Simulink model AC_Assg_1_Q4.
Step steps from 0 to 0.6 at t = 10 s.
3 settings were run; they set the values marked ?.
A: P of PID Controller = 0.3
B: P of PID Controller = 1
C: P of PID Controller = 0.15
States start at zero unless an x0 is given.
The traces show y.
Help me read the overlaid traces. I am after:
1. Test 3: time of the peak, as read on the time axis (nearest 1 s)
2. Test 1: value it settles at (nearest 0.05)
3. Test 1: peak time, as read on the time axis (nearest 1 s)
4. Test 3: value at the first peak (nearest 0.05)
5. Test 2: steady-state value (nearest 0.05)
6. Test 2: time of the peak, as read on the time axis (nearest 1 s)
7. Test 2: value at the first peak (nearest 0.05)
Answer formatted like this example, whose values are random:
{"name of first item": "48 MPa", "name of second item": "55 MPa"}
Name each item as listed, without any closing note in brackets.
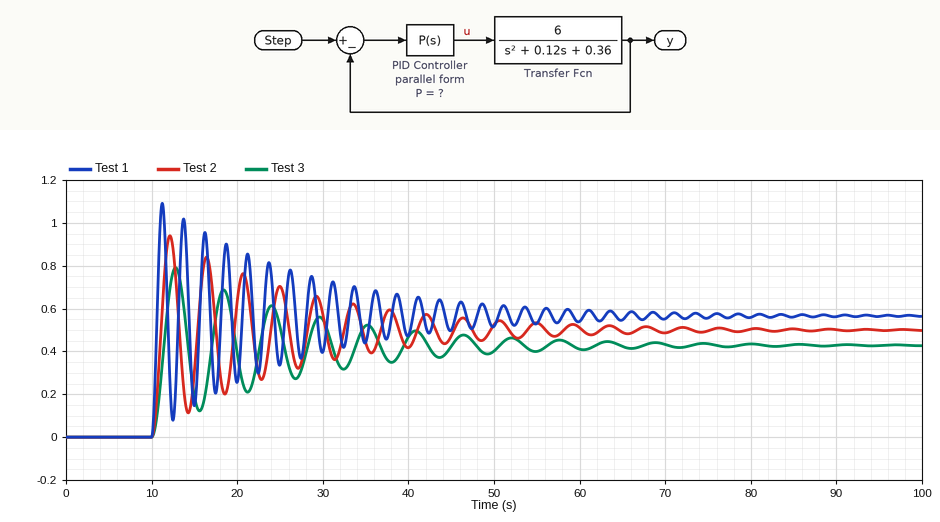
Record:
{"Test 3: time of the peak, as read on the time axis": "13 s", "Test 1: value it settles at": "0.55", "Test 1: peak time, as read on the time axis": "11 s", "Test 3: value at the first peak": "0.80", "Test 2: steady-state value": "0.50", "Test 2: time of the peak, as read on the time axis": "12 s", "Test 2: value at the first peak": "0.95"}
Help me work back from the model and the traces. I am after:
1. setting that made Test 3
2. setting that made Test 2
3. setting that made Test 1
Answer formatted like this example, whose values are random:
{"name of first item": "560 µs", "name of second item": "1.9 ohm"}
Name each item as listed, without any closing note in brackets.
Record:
{"setting that made Test 3": "C", "setting that made Test 2": "A", "setting that made Test 1": "B"}
